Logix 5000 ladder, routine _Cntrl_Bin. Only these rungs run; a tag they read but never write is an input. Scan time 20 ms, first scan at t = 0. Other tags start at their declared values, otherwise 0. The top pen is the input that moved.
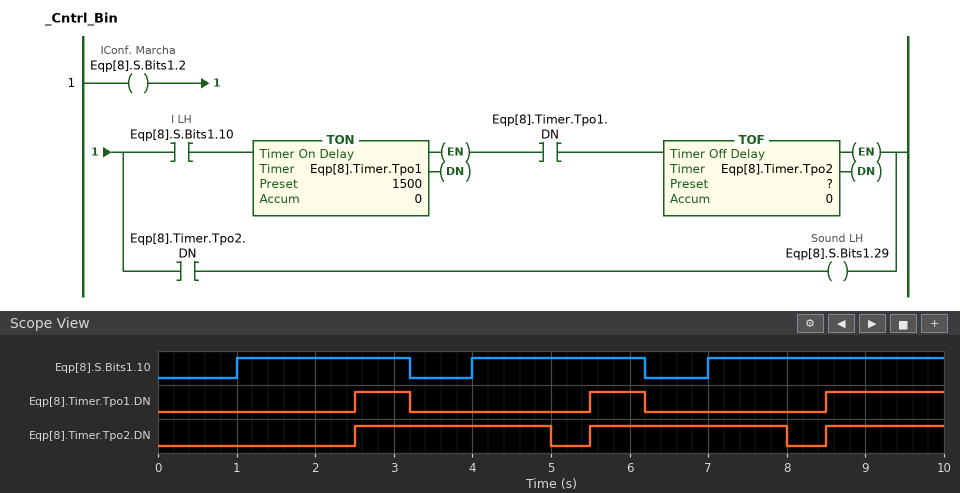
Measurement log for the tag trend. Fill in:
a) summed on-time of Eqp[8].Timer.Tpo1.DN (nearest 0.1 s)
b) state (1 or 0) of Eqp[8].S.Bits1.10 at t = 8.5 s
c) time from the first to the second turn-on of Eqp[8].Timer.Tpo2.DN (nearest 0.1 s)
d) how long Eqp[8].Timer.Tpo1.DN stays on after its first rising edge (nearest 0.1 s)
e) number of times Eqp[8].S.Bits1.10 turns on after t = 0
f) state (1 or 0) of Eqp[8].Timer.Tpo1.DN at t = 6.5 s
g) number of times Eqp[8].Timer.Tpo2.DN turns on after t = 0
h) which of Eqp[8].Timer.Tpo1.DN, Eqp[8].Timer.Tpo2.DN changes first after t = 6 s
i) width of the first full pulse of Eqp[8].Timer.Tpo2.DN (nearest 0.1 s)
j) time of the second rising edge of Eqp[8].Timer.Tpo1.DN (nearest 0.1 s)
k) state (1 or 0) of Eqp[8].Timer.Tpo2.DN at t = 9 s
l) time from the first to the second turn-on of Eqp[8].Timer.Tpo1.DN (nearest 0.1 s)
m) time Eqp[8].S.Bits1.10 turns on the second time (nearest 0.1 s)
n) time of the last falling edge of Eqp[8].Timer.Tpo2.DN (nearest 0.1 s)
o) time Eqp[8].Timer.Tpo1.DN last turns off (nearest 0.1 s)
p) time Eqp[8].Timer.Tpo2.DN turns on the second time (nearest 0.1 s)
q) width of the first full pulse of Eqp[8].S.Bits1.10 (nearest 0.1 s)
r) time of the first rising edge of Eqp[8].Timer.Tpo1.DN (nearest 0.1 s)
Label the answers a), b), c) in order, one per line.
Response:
a) 2.9 s
b) 1
c) 3.0 s
d) 0.7 s
e) 3
f) 0
g) 3
h) Eqp[8].Timer.Tpo1.DN
i) 2.5 s
j) 5.5 s
k) 1
l) 3.0 s
m) 4.0 s
n) 8.0 s
o) 6.2 s
p) 5.5 s
q) 2.2 s
r) 2.5 s
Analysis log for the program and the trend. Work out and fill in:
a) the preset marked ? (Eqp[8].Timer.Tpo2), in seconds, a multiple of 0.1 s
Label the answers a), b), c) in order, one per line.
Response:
a) 1.8 s
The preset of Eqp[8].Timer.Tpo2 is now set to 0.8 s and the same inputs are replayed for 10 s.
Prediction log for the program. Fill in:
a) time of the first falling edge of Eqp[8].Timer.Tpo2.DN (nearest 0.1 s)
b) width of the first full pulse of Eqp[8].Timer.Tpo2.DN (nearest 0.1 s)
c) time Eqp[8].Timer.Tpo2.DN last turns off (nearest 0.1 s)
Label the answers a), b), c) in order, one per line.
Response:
a) 4.0 s
b) 1.5 s
c) 7.0 s
